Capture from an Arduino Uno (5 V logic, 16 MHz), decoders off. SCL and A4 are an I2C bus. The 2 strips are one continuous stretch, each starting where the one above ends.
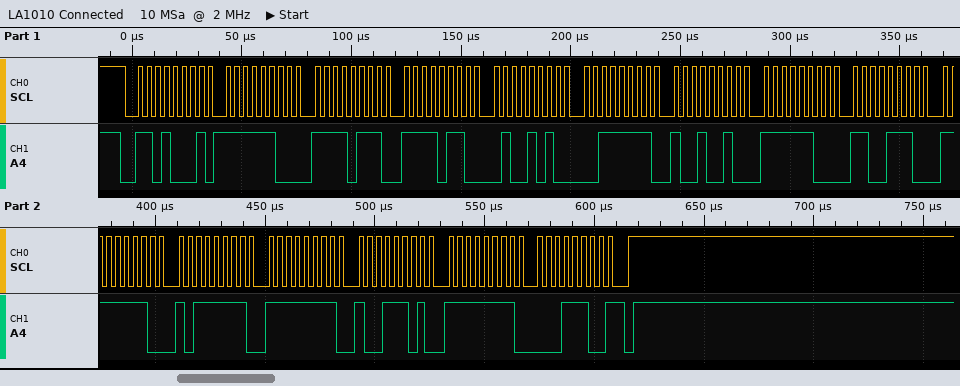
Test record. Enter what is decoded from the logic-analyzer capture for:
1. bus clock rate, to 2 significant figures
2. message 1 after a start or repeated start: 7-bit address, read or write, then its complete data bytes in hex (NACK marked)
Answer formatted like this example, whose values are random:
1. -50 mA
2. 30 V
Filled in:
1. 250 kHz
2. 0x68 read: FC F7 F6 4A 3F 92 FC CE FE BF FF 9D FF 1C NACK
